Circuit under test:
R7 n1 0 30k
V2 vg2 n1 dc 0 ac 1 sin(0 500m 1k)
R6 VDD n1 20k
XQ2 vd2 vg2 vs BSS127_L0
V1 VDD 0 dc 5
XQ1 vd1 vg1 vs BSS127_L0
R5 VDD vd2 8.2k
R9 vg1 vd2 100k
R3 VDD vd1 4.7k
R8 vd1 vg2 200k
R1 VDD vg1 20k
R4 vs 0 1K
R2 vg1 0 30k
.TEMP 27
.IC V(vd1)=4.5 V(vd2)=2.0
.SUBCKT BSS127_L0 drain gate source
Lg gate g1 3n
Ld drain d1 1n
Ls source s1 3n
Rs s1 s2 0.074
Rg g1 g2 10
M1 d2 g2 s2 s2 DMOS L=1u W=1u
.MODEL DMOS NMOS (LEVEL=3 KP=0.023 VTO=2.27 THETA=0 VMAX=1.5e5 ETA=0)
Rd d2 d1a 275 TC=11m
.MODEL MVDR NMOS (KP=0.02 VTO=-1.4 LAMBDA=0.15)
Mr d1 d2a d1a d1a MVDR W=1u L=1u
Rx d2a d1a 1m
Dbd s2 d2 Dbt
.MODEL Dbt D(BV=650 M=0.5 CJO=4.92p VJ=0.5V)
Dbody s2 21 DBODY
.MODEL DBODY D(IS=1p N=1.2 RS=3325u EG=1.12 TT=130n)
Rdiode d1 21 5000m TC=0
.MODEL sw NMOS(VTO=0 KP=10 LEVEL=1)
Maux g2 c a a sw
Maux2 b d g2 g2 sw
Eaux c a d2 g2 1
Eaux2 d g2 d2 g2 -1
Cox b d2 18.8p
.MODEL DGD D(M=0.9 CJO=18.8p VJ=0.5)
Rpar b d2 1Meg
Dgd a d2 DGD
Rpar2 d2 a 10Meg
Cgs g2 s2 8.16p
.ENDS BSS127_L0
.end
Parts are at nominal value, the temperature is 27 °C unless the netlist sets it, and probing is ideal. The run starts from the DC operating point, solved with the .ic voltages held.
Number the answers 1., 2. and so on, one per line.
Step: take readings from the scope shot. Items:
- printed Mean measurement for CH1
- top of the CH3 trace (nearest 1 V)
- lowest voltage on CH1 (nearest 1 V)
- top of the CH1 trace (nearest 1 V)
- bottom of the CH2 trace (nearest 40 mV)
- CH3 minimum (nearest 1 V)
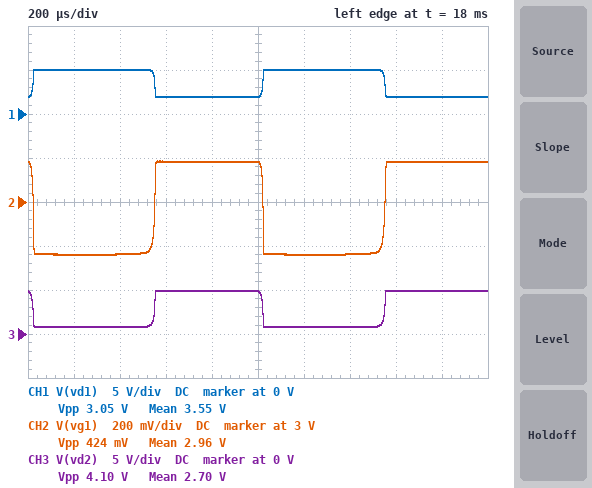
1. 3.55 V
2. 5 V
3. 2 V
4. 5 V
5. 2.76 V
6. 1 V
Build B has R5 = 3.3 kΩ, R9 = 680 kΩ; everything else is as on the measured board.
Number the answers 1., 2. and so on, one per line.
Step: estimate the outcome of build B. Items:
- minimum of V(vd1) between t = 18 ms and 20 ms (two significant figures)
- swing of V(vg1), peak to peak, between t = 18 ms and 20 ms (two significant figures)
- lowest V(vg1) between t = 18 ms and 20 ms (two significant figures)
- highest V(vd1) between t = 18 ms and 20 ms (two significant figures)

1. 2.5 V
2. 50 mV
3. 3.0 V
4. 5.0 V
